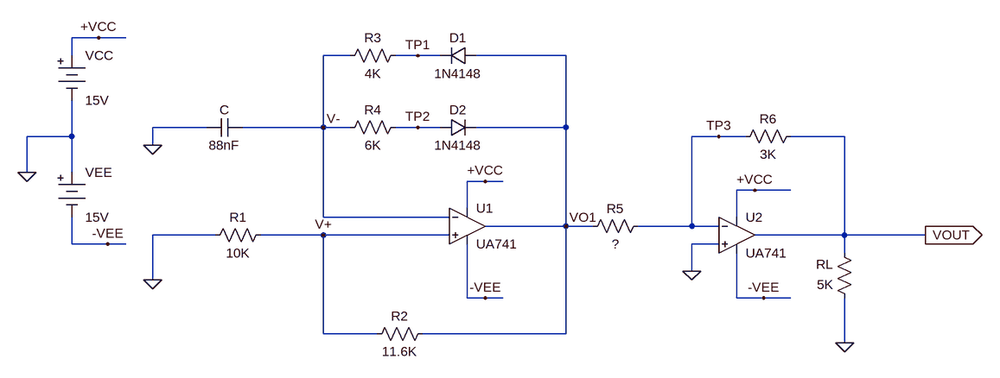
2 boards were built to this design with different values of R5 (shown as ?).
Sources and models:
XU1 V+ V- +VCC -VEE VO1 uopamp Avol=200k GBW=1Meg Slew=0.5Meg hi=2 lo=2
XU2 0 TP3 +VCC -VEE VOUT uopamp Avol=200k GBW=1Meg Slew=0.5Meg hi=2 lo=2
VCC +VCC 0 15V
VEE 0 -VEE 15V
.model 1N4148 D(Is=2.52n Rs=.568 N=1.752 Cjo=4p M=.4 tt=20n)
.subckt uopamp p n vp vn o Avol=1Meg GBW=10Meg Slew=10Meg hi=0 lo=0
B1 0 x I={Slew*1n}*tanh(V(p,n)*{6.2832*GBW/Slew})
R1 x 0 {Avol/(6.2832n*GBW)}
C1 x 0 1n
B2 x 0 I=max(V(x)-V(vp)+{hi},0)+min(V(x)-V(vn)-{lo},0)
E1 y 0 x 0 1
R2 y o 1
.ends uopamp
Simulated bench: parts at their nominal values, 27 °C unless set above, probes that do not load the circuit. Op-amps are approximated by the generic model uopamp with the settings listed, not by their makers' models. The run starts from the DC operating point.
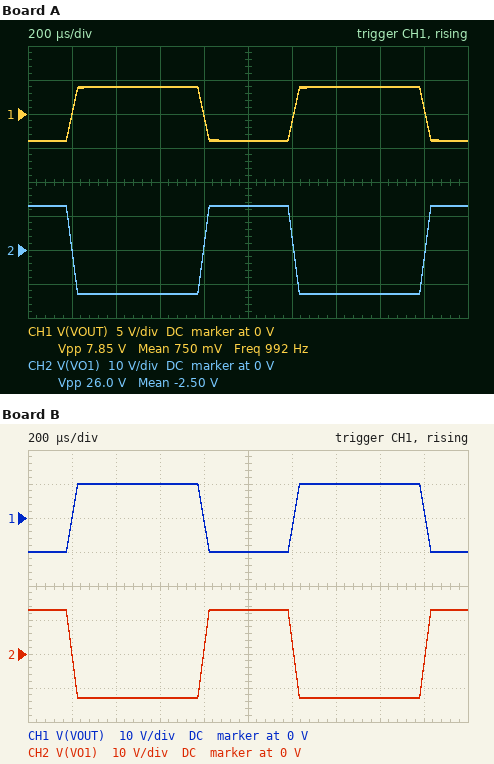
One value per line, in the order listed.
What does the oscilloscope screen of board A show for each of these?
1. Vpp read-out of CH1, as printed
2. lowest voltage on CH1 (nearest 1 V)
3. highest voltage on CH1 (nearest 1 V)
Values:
7.85 V
-4 V
4 V
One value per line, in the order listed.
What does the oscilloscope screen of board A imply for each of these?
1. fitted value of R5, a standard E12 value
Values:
10 kΩ
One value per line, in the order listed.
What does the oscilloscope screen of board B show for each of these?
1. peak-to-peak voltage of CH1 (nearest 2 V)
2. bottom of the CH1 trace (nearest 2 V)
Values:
20 V
-10 V
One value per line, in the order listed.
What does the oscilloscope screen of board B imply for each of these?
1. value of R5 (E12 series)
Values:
3.9 kΩ
